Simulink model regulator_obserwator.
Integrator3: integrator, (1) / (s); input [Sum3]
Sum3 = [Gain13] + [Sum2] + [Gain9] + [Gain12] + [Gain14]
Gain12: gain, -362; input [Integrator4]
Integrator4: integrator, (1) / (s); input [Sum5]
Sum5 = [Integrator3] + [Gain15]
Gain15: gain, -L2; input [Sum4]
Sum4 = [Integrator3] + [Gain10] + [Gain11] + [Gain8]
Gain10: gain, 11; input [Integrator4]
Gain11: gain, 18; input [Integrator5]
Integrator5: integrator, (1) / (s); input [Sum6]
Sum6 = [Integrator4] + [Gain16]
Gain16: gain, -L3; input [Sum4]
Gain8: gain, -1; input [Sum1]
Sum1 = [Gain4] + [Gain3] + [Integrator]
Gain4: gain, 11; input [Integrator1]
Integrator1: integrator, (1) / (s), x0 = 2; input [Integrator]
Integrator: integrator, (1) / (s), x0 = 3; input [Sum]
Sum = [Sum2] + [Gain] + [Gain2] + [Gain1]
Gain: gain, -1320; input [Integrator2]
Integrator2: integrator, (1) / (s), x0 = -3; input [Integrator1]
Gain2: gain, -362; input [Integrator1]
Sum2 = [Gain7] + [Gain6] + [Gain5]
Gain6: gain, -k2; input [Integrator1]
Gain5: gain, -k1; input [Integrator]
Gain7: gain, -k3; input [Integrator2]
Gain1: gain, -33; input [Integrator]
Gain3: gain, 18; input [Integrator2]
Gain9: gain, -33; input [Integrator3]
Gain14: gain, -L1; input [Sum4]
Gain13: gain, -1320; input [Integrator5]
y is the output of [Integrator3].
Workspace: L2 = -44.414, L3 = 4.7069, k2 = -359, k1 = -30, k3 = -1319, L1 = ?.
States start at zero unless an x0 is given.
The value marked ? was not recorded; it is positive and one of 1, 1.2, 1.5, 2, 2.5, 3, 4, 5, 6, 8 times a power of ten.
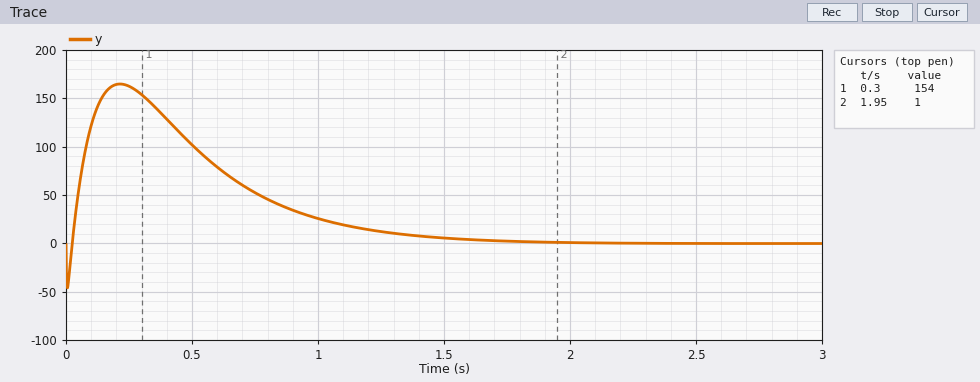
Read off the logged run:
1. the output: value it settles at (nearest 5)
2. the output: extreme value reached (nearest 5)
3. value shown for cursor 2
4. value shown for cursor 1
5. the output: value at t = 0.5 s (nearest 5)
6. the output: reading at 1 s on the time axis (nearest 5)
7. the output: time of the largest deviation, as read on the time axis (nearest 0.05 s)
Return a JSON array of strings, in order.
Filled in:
["0", "165", "1", "154", "100", "25", "0.20 s"]
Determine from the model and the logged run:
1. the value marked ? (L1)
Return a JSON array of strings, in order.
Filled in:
["800"]
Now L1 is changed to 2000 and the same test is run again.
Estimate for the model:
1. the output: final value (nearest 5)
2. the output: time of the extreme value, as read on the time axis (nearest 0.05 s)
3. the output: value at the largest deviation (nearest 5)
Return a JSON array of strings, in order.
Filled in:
["0", "0.25 s", "50"]
